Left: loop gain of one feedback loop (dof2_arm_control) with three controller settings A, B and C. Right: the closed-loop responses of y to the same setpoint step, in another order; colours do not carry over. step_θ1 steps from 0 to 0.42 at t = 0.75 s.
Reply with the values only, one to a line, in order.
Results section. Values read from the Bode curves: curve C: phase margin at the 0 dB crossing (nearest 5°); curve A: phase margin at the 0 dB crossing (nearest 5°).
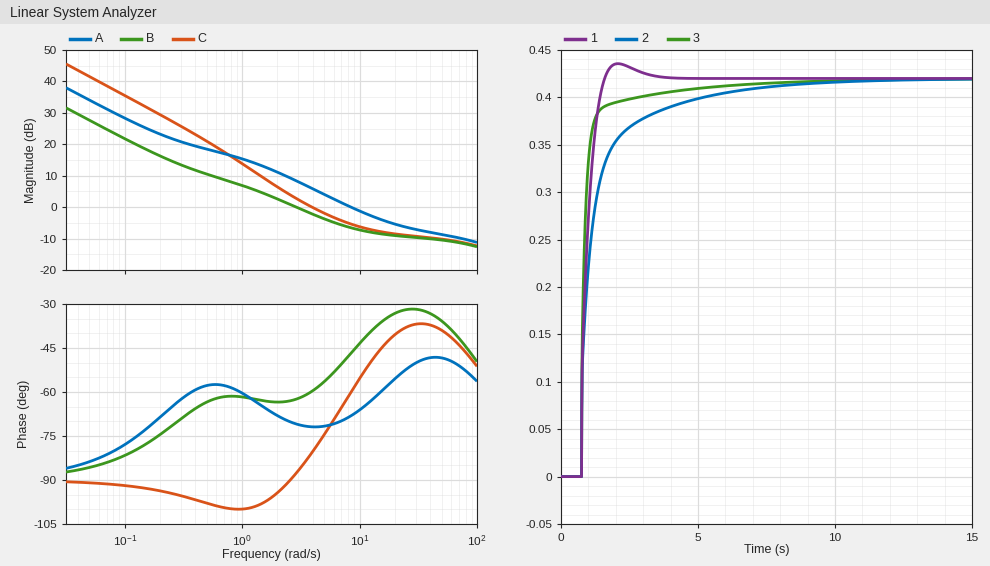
100°
110°
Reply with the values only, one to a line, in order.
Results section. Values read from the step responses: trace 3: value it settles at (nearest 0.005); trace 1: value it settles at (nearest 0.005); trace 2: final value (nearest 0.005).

0.420
0.420
0.420
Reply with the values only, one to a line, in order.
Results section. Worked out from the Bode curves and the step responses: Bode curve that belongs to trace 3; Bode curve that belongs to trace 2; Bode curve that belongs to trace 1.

A
B
C
